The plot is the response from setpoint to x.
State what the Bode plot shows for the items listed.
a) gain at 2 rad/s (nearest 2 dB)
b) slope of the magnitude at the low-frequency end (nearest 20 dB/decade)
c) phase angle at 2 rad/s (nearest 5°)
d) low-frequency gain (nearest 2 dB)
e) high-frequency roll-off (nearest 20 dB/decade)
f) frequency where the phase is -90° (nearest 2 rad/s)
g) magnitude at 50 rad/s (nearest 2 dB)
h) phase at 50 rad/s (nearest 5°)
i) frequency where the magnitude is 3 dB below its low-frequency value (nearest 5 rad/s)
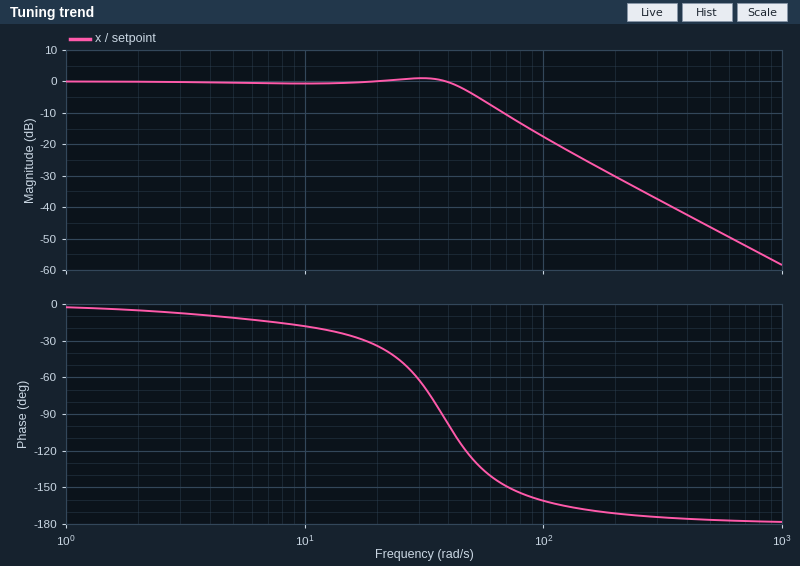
0 dB
0 dB/decade
-5°
0 dB
-40 dB/decade
38 rad/s
-4 dB
-125°
50 rad/s
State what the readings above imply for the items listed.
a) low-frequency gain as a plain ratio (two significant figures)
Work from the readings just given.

1.0
